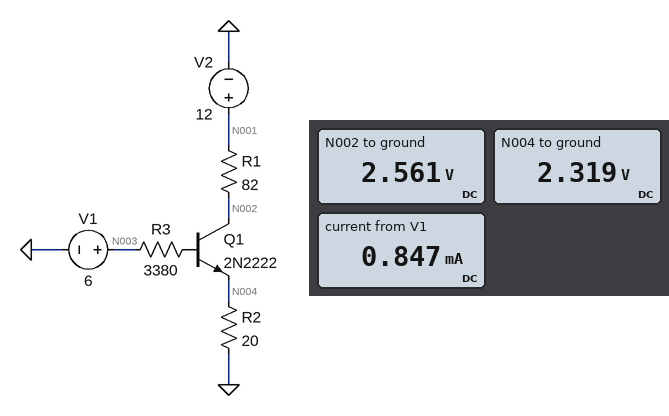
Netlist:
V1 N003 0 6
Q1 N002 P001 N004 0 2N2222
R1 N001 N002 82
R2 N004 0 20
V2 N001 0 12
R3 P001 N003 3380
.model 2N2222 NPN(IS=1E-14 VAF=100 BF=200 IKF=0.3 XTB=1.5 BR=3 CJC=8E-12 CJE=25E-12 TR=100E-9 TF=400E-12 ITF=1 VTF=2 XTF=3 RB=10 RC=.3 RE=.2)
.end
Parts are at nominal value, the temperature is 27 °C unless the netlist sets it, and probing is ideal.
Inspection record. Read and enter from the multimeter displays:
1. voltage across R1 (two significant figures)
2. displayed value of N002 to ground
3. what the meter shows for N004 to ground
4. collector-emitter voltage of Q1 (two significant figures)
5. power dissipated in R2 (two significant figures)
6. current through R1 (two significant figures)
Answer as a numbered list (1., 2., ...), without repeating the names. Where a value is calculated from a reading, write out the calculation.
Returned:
1. 12 V - 2.561 V = 9.4 V
2. 2.561 V
3. 2.319 V
4. 2.561 V - 2.319 V = 240 mV
5. (2.319 V)^2 / 20 Ω = 270 mW
6. (12 V - 2.561 V) / 82 Ω = 120 mA
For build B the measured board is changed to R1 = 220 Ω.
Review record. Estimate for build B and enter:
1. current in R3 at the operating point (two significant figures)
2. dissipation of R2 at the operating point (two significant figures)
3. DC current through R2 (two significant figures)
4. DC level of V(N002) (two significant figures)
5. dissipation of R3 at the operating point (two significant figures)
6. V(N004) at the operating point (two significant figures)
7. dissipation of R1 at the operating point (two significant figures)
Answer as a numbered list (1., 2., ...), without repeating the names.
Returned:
1. 1.2 mA
2. 51 mW
3. 51 mA
4. 1.1 V
5. 5.2 mW
6. 1.0 V
7. 540 mW
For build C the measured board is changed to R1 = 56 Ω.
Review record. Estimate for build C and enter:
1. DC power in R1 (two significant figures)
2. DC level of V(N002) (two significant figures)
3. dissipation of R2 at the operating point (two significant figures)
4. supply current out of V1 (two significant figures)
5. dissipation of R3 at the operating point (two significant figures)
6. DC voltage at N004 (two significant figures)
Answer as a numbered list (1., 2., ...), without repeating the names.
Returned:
1. 810 mW
2. 5.3 V
3. 290 mW
4. 820 µA
5. 2.3 mW
6. 2.4 V
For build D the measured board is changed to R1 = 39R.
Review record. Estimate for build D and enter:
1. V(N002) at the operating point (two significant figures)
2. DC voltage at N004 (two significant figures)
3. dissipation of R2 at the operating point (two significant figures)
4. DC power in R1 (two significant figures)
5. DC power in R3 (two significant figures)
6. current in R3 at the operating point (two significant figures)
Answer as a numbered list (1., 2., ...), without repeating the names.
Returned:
1. 7.3 V
2. 2.4 V
3. 300 mW
4. 570 mW
5. 2.2 mW
6. 810 µA
